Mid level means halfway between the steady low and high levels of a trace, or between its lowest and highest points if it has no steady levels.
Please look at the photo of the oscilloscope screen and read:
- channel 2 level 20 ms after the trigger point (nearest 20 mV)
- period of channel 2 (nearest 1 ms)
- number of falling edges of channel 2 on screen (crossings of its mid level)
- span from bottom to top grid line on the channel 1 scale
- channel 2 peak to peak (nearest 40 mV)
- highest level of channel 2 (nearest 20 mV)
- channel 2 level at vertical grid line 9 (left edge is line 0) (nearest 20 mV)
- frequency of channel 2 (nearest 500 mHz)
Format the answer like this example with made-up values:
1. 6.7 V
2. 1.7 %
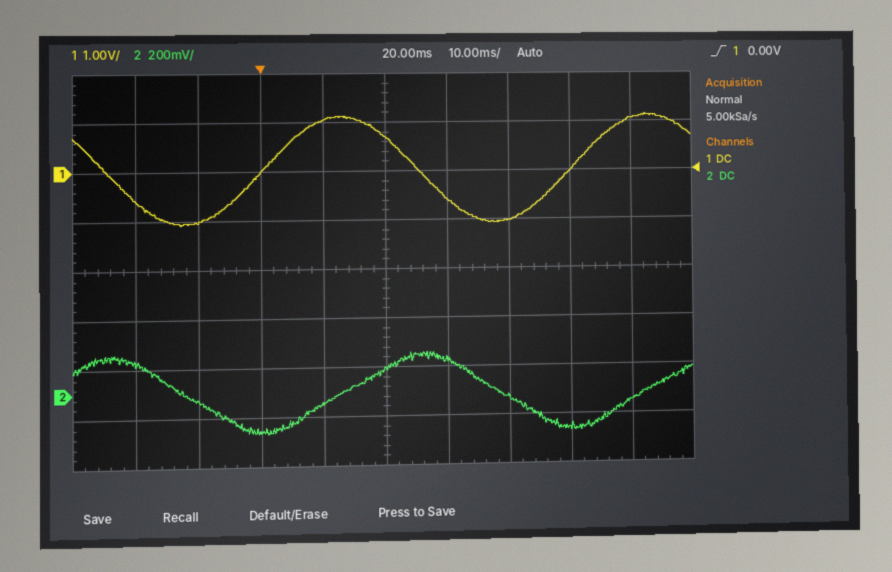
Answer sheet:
1. 100 mV
2. 50 ms
3. 2
4. 8 V
5. 320 mV
6. 160 mV
7. -40 mV
8. 20.0 Hz
